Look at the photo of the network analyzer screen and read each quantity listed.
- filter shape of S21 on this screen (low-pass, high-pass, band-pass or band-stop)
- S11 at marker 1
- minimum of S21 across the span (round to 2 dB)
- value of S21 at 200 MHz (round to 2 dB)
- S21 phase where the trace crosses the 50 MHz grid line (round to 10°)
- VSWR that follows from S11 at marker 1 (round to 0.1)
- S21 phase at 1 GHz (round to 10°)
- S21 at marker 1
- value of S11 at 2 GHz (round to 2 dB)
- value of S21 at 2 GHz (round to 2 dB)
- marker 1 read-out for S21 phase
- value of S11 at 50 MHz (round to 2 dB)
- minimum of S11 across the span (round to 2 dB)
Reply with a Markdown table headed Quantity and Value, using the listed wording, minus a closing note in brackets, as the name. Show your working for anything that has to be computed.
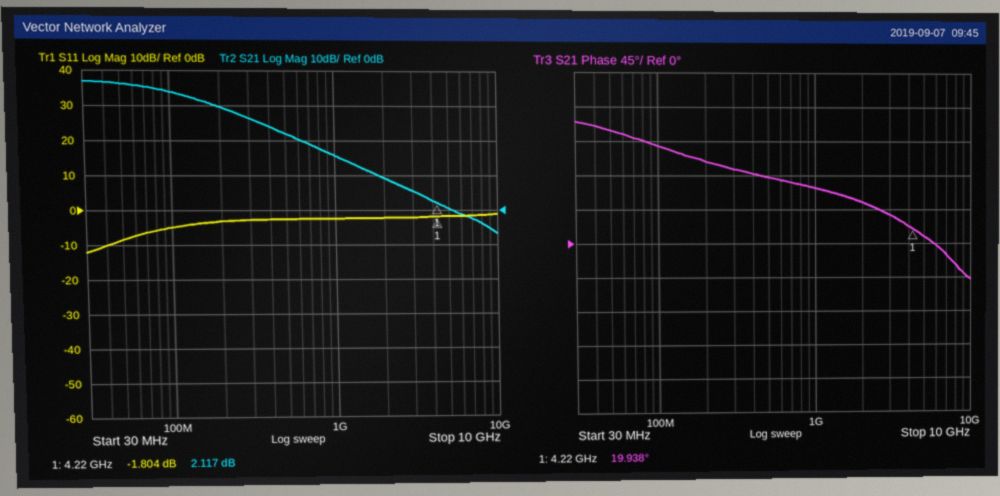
| Quantity | Value |
|---|---|
| filter shape of S21 on this screen | low-pass |
| S11 at marker 1 | -1.804 dB |
| minimum of S21 across the span | -6 dB |
| value of S21 at 200 MHz | 30 dB |
| S21 phase where the trace crosses the 50 MHz grid line | 150° |
| VSWR that follows from S11 at marker 1 | (1 + 0.8125)/(1 − 0.8125) ≈ 9.7 |
| S21 phase at 1 GHz | 70° |
| S21 at marker 1 | 2.117 dB |
| value of S11 at 2 GHz | -2 dB |
| value of S21 at 2 GHz | 10 dB |
| marker 1 read-out for S21 phase | 19.938° |
| value of S11 at 50 MHz | -8 dB |
| minimum of S11 across the span | -12 dB |
